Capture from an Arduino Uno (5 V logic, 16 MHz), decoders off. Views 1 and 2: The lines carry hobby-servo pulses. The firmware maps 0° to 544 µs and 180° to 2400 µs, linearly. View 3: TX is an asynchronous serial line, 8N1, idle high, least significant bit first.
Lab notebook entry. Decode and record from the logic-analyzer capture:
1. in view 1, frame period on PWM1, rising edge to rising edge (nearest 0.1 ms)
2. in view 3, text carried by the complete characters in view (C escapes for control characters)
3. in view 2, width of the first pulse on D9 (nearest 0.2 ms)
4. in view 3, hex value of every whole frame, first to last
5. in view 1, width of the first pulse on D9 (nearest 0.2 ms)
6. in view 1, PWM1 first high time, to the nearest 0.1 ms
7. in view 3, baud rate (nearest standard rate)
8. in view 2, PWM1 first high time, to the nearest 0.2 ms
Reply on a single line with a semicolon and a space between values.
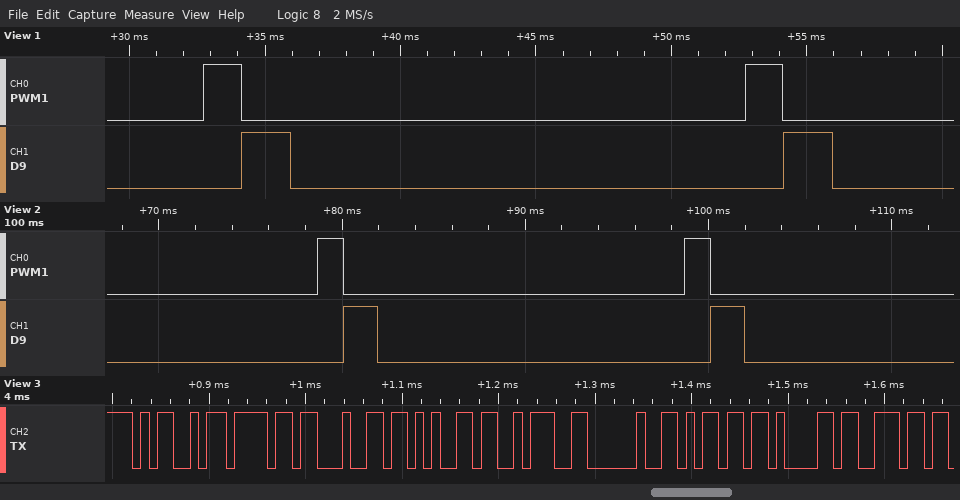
20.0 ms; "Mode: man"; 1.8 ms; 4D 6F 64 65 3A 20 6D 61 6E; 1.8 ms; 1.4 ms; 115200 baud; 1.4 ms
